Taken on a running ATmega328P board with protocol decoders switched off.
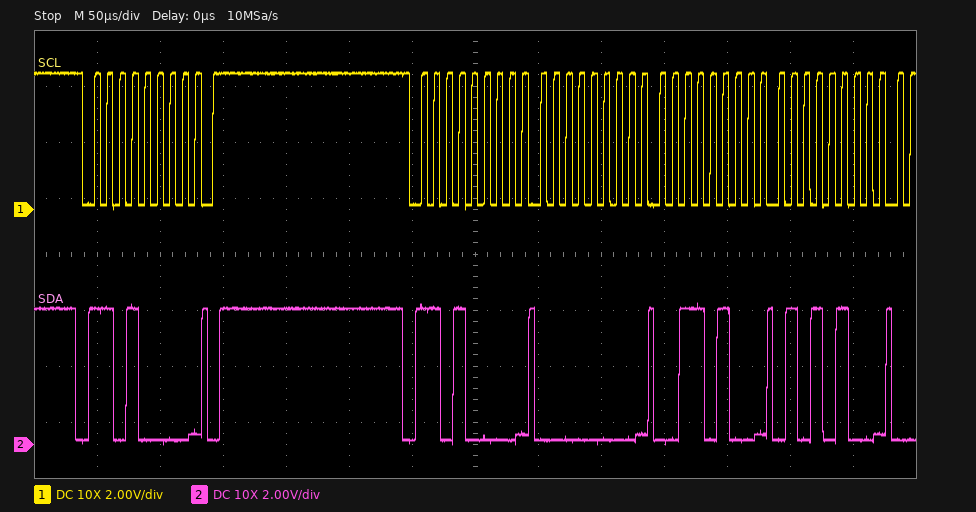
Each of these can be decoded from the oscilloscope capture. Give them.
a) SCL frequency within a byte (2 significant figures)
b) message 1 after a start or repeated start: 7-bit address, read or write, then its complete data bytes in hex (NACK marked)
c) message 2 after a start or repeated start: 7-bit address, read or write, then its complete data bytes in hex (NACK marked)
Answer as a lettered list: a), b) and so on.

a) 100 kHz
b) 0x68 write
c) 0x68 write: 00 34 54
